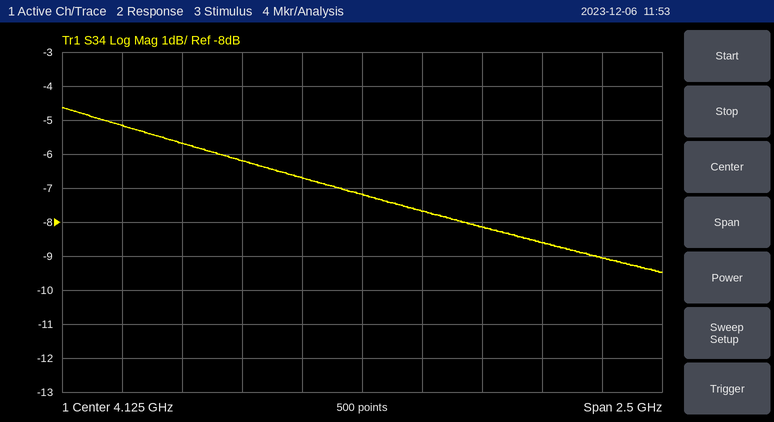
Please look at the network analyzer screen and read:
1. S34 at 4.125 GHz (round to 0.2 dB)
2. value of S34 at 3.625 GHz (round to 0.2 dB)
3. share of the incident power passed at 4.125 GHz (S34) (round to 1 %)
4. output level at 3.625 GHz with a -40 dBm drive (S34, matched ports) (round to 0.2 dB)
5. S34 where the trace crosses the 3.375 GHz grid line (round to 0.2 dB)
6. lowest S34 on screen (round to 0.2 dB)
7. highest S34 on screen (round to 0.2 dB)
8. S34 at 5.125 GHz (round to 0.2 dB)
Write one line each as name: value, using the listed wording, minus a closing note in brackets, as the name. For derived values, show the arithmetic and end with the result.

S34 at 4.125 GHz: -7.2 dB
value of S34 at 3.625 GHz: -6.2 dB
share of the incident power passed at 4.125 GHz (S34): 10^(-7.2/10) ≈ 19 %
output level at 3.625 GHz with a -40 dBm drive (S34, matched ports): -40 dBm + (-6.2 dB) = -46.2 dBm
S34 where the trace crosses the 3.375 GHz grid line: -5.6 dB
lowest S34 on screen: -9.4 dB
highest S34 on screen: -4.6 dB
S34 at 5.125 GHz: -9.0 dB
